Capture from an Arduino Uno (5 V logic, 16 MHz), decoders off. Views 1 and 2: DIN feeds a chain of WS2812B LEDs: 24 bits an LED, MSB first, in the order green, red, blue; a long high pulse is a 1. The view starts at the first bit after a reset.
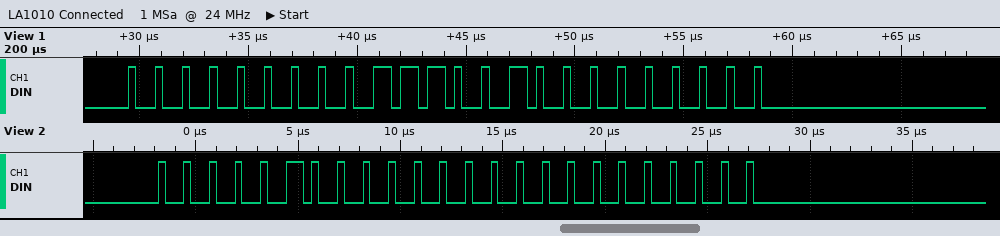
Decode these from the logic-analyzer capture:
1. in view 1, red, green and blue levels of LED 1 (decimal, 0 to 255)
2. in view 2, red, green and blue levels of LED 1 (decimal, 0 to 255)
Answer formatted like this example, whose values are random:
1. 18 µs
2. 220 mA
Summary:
1. 114, 0, 0
2. 0, 4, 0
